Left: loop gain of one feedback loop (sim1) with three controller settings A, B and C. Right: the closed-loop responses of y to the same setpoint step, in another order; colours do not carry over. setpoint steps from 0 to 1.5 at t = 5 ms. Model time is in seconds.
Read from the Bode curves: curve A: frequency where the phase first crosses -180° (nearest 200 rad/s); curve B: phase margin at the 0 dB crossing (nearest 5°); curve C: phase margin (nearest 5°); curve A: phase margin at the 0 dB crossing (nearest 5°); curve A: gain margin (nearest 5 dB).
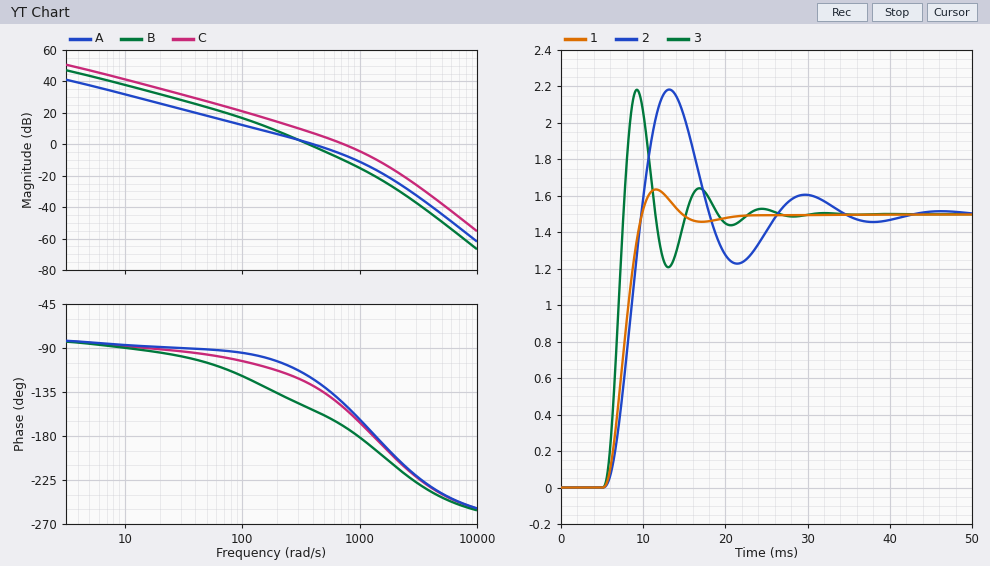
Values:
1400 rad/s
30°
30°
60°
15 dB
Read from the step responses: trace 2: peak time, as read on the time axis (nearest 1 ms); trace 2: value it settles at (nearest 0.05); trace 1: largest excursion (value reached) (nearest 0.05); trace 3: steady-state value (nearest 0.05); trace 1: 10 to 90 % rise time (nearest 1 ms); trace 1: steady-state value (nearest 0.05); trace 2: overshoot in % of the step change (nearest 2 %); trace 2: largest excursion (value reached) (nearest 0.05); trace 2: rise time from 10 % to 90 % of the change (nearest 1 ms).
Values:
13 ms
1.50
1.65
1.50
3 ms
1.50
46 %
2.20
3 ms
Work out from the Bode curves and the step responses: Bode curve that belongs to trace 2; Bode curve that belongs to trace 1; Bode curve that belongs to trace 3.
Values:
B
A
C
